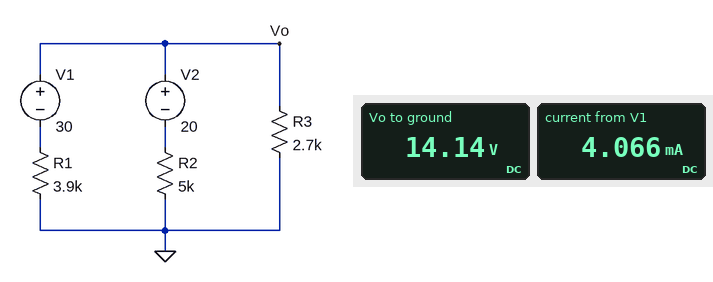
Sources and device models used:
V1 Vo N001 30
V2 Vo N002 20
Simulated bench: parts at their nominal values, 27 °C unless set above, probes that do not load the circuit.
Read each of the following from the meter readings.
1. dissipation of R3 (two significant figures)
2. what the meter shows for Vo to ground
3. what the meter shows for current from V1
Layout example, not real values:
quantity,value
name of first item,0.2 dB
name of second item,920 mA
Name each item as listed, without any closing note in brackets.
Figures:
quantity,value
dissipation of R3,74 mW
what the meter shows for Vo to ground,14.14 V
what the meter shows for current from V1,4.066 mA
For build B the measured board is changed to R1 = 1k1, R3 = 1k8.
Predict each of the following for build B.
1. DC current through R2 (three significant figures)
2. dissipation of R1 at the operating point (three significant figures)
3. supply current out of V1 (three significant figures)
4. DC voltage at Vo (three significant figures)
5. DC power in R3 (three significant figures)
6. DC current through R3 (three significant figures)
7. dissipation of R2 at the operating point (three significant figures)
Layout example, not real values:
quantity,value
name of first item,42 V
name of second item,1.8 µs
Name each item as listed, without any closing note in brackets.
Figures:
quantity,value
DC current through R2,243 µA
dissipation of R1 at the operating point,114 mW
supply current out of V1,10.2 mA
DC voltage at Vo,18.8 V
DC power in R3,196 mW
DC current through R3,10.4 mA
dissipation of R2 at the operating point,295 µW
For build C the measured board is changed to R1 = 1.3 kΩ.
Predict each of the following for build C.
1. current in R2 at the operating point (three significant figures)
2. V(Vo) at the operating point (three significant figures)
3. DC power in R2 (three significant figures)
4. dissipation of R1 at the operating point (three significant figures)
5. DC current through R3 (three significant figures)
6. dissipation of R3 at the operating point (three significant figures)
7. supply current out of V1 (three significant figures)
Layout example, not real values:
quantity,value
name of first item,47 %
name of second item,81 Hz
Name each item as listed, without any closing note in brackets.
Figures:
quantity,value
current in R2 at the operating point,42.5 µA
V(Vo) at the operating point,20.2 V
DC power in R2,9.05 µW
dissipation of R1 at the operating point,73.7 mW
DC current through R3,7.49 mA
dissipation of R3 at the operating point,151 mW
supply current out of V1,7.53 mA
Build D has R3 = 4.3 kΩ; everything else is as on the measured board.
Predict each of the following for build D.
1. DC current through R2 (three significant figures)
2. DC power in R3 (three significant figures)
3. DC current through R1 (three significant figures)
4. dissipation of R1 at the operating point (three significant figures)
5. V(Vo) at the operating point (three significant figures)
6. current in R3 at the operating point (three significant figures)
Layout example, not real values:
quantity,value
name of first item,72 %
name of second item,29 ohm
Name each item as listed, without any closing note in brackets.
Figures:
quantity,value
DC current through R2,606 µA
DC power in R3,67.0 mW
DC current through R1,3.34 mA
dissipation of R1 at the operating point,43.5 mW
V(Vo) at the operating point,17.0 V
current in R3 at the operating point,3.95 mA
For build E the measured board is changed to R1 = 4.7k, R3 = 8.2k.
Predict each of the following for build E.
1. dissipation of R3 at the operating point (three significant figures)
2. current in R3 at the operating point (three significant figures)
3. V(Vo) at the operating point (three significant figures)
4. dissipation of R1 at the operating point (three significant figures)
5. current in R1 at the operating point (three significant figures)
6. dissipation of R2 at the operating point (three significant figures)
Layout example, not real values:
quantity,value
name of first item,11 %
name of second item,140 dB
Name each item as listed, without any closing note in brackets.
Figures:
quantity,value
dissipation of R3 at the operating point,46.0 mW
current in R3 at the operating point,2.37 mA
V(Vo) at the operating point,19.4 V
dissipation of R1 at the operating point,23.8 mW
current in R1 at the operating point,2.25 mA
dissipation of R2 at the operating point,67.8 µW
